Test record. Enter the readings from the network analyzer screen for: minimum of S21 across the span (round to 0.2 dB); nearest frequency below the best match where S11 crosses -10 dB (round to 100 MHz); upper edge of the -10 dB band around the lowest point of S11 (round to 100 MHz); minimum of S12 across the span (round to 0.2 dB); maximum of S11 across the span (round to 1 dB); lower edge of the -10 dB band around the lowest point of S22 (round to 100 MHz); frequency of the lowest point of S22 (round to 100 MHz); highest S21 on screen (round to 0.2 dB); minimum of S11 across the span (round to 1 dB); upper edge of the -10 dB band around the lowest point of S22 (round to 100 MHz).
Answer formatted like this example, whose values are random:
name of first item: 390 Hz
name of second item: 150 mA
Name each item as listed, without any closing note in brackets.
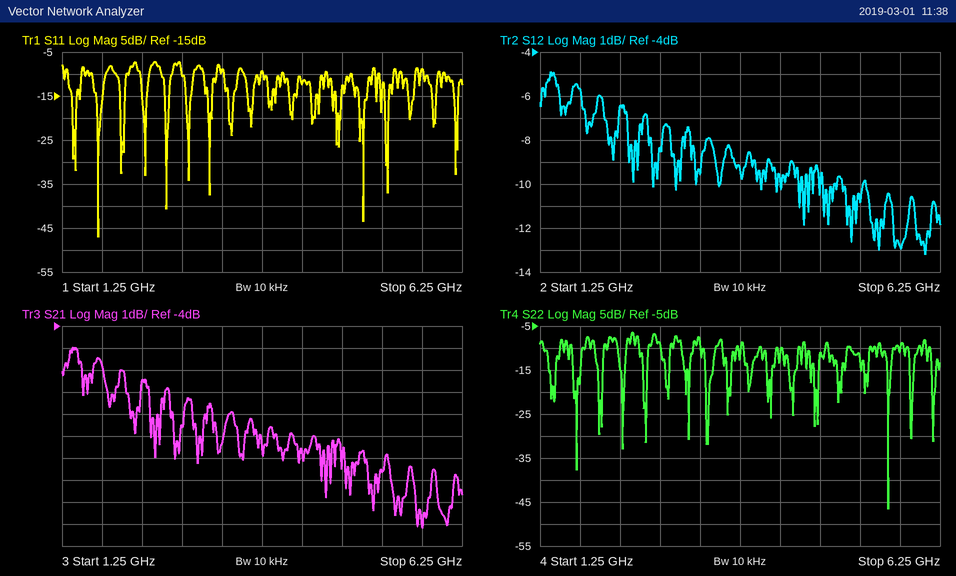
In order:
minimum of S21 across the span: -13.2 dB
nearest frequency below the best match where S11 crosses -10 dB: 1.6 GHz
upper edge of the -10 dB band around the lowest point of S11: 1.8 GHz
minimum of S12 across the span: -13.2 dB
maximum of S11 across the span: -7 dB
lower edge of the -10 dB band around the lowest point of S22: 5.5 GHz
frequency of the lowest point of S22: 5.6 GHz
highest S21 on screen: -5.0 dB
minimum of S11 across the span: -47 dB
upper edge of the -10 dB band around the lowest point of S22: 5.7 GHz
